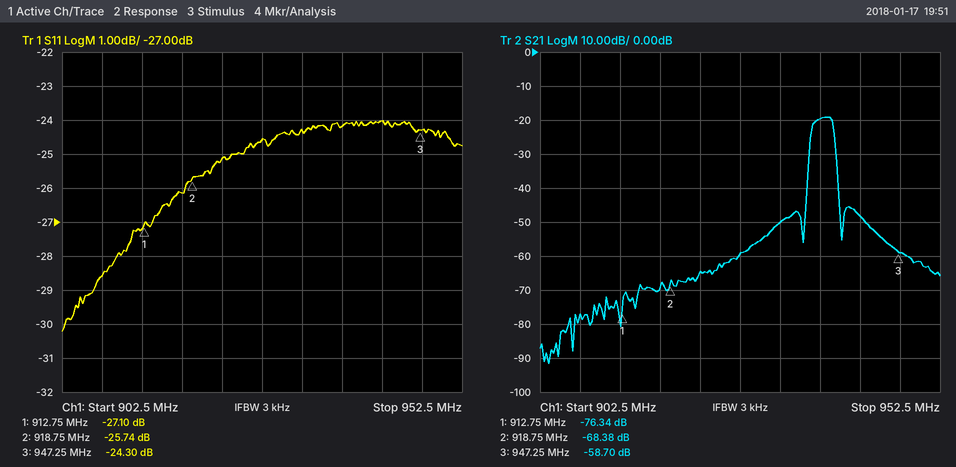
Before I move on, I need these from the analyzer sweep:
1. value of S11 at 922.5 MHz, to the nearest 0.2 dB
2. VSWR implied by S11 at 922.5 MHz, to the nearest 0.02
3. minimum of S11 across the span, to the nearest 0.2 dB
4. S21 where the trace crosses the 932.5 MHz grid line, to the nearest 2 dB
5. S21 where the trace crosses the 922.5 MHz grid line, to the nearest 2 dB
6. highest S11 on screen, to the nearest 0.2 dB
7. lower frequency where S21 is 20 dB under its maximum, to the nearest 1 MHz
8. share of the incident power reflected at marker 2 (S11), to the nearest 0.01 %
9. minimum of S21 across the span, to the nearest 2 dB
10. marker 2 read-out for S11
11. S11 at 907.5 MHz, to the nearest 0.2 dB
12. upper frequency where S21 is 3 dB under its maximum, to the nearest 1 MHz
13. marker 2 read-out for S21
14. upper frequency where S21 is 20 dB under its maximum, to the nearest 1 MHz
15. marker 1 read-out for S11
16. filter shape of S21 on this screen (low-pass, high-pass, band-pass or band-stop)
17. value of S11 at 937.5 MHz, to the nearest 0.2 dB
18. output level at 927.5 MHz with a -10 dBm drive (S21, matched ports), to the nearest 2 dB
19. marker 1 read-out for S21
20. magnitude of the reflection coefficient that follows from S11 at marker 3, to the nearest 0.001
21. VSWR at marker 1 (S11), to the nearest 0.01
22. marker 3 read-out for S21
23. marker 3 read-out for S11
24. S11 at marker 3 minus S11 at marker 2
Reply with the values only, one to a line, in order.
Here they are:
-25.2 dB
1.12
-30.2 dB
-50 dB
-64 dB
-24.0 dB
936 MHz
0.27 %
-92 dB
-25.74 dB
-28.6 dB
939 MHz
-68.38 dB
940 MHz
-27.10 dB
band-pass
-24.2 dB
-70 dBm
-76.34 dB
0.061
1.09
-58.70 dB
-24.30 dB
1.44 dB
